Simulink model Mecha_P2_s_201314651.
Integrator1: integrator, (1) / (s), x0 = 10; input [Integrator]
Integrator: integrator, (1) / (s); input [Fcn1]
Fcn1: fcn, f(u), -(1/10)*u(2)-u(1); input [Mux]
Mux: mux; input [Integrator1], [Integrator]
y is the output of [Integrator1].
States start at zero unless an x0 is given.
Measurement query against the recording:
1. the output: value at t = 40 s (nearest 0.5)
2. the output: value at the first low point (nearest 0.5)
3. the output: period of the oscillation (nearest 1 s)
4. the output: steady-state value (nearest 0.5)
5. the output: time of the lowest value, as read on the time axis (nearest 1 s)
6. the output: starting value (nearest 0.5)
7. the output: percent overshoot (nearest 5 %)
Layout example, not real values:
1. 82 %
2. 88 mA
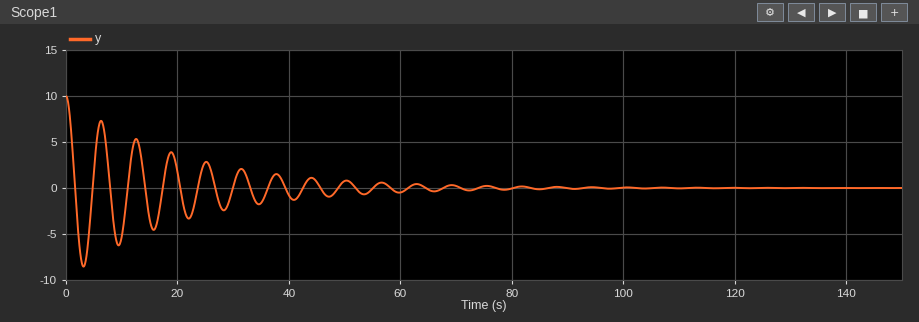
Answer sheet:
1. -1.0
2. -8.5
3. 6 s
4. 0.0
5. 3 s
6. 10.0
7. 85 %
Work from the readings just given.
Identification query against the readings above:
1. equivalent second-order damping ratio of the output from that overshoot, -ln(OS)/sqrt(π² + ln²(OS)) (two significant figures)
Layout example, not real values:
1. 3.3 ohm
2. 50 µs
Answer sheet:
1. 0.052
